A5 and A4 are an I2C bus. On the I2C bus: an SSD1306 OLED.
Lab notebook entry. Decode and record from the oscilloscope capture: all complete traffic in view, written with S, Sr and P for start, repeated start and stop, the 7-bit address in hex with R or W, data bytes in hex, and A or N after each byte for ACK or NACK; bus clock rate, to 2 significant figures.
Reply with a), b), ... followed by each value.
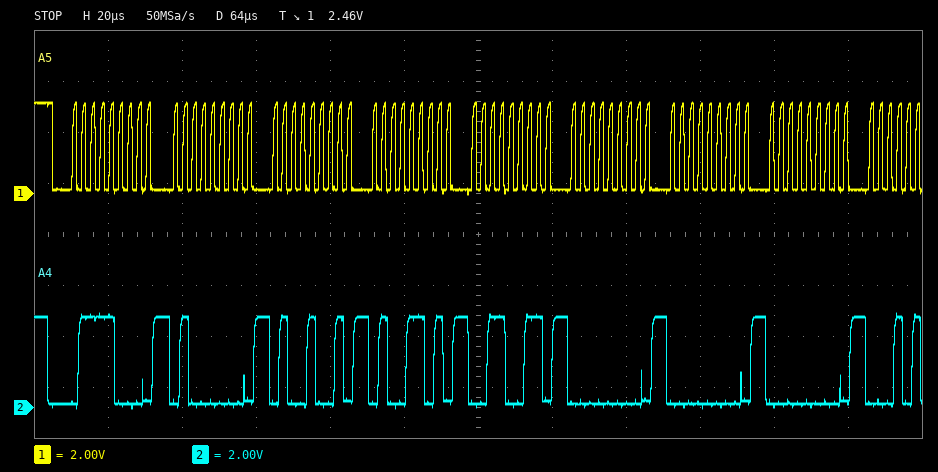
a) S 3CW A 40 A 49 A 4D A 33 A 00 A 00 A 00 A
b) 400 kHz
